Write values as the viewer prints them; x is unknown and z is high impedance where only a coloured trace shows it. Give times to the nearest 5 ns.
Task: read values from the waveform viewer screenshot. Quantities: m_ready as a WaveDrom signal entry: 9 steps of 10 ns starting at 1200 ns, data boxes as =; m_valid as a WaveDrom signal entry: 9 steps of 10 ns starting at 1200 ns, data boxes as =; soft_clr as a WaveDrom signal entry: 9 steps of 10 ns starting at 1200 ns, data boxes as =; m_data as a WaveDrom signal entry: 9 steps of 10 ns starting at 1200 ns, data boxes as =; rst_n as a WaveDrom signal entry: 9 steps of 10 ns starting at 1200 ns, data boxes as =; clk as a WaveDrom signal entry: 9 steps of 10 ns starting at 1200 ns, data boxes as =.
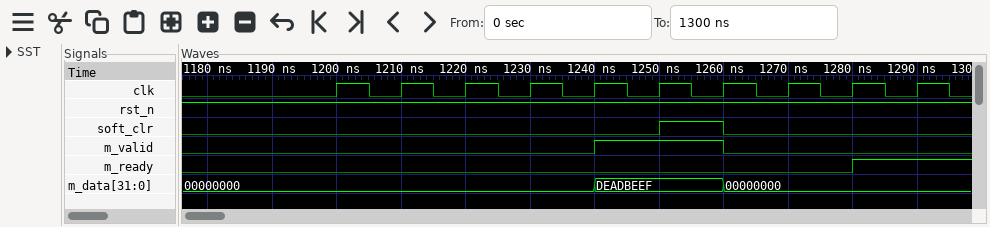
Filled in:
{name: 'm_ready', wave: '0.......1'}
{name: 'm_valid', wave: '0...1.0..'}
{name: 'soft_clr', wave: '0....10..'}
{name: 'm_data', wave: '=...=.=..', data: '00000000 DEADBEEF 00000000'}
{name: 'rst_n', wave: '1........'}
{name: 'clk', wave: 'p........'}
